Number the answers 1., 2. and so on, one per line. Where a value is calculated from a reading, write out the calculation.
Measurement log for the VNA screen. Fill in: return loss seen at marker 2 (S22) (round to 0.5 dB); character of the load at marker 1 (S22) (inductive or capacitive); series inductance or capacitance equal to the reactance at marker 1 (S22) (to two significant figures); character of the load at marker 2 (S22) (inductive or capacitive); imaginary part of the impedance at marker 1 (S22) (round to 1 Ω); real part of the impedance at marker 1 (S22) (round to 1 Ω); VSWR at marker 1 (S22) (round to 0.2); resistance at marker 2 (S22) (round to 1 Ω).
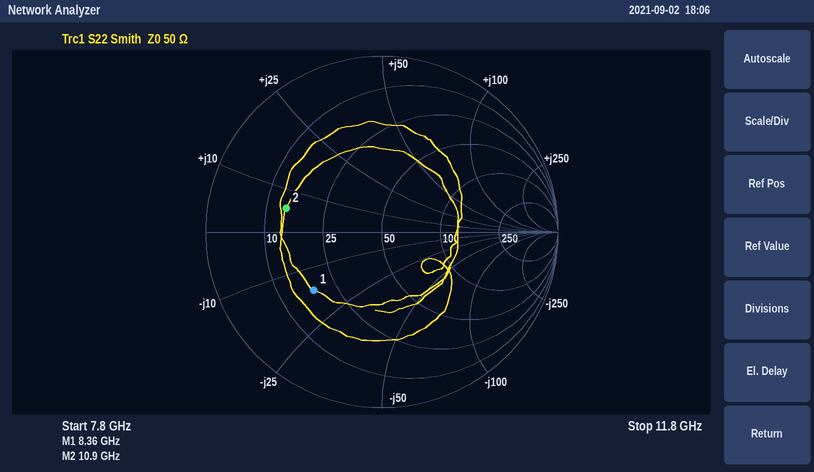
1. 5.0 dB
2. capacitive
3. C = 1/(2π × 8.36 GHz × 16 Ω) ≈ 1.2 pF
4. inductive
5. -16 Ω
6. 18 Ω
7. 3.0
8. 14 Ω
